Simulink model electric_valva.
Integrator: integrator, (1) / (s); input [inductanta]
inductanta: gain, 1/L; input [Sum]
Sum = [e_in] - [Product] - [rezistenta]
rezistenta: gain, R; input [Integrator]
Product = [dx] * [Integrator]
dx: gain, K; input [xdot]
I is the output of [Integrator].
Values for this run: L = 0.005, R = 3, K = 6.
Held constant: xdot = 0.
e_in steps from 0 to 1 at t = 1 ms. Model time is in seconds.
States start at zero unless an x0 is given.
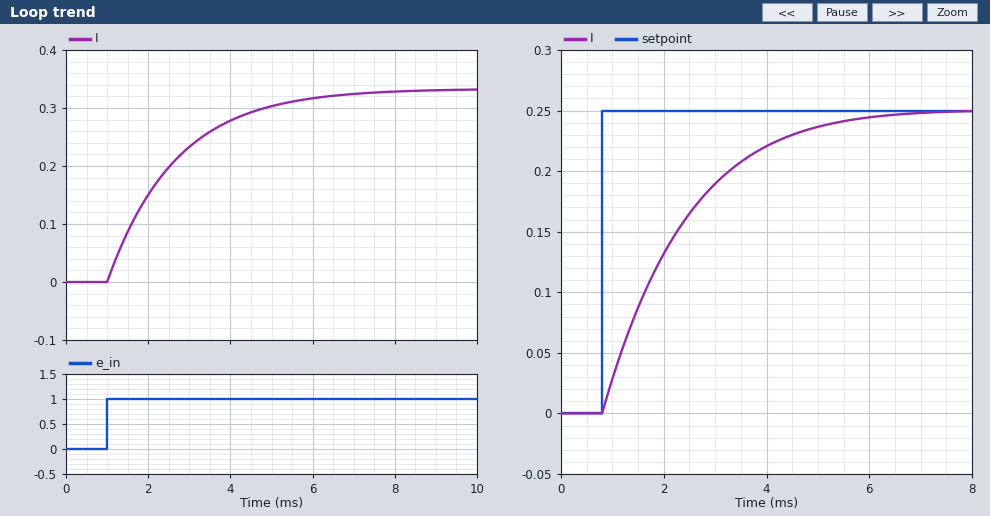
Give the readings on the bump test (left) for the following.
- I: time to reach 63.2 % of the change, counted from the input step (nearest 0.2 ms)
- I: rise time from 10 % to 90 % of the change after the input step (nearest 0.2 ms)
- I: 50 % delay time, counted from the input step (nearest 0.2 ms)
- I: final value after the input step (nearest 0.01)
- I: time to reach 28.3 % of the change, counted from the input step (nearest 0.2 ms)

1.6 ms
3.6 ms
1.2 ms
0.33
0.6 ms
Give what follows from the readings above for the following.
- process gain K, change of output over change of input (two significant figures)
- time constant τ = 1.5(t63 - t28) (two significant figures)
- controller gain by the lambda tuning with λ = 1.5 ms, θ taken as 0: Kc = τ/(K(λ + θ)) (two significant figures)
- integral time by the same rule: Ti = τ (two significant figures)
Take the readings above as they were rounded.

0.33
1.5 ms
3.0
1.5 ms
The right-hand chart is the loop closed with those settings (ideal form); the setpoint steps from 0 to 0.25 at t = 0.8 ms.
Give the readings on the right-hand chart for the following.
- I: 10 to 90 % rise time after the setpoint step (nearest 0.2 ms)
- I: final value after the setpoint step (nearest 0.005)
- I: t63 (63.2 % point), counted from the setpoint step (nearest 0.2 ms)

3.2 ms
0.250
1.6 ms
